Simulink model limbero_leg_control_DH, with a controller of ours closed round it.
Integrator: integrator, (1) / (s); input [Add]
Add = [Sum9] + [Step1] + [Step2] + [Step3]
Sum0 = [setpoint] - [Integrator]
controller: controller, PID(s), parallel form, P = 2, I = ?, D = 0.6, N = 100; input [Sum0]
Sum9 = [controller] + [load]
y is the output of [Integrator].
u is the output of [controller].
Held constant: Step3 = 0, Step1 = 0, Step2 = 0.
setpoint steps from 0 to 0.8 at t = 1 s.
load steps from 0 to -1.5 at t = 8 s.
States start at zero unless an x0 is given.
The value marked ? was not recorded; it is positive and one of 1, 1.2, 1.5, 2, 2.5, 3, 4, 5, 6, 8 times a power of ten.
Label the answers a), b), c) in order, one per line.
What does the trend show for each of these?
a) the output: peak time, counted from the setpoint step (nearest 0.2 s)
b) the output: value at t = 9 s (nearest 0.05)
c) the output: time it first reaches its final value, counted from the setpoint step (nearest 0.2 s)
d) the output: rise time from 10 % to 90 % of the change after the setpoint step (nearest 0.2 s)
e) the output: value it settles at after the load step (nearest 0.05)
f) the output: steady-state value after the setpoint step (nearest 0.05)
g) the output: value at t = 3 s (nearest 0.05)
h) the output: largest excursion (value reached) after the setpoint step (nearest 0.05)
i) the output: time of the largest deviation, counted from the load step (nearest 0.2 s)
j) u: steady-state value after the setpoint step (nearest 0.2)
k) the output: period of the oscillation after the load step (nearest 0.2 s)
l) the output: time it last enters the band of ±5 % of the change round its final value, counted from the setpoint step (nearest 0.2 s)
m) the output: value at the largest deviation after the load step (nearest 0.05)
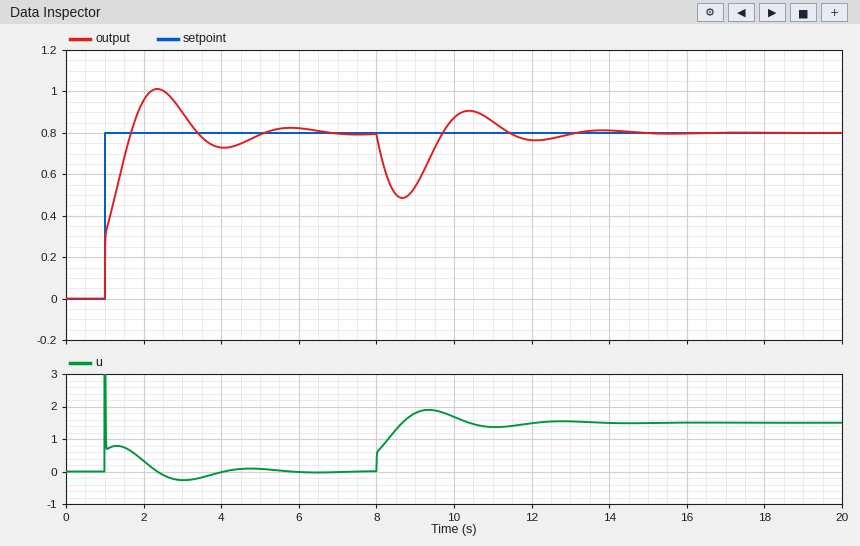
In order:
a) 1.4 s
b) 0.55
c) 0.6 s
d) 0.6 s
e) 0.80
f) 0.80
g) 0.90
h) 1.00
i) 0.6 s
j) 0.0
k) 3.4 s
l) 3.6 s
m) 0.50
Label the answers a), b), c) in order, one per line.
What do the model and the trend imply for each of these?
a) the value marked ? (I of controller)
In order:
a) 6
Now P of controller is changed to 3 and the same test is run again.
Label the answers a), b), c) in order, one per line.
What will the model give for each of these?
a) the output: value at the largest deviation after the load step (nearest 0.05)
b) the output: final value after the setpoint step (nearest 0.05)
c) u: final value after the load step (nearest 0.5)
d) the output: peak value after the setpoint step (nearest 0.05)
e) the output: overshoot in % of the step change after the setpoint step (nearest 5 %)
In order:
a) 0.55
b) 0.80
c) 1.5
d) 0.95
e) 20 %
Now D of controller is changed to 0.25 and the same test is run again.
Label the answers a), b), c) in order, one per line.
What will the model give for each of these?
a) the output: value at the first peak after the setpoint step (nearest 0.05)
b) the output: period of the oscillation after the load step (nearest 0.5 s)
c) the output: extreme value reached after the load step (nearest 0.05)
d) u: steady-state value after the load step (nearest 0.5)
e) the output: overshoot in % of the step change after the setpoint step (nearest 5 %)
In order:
a) 1.05
b) 3.0 s
c) 0.45
d) 1.5
e) 30 %
